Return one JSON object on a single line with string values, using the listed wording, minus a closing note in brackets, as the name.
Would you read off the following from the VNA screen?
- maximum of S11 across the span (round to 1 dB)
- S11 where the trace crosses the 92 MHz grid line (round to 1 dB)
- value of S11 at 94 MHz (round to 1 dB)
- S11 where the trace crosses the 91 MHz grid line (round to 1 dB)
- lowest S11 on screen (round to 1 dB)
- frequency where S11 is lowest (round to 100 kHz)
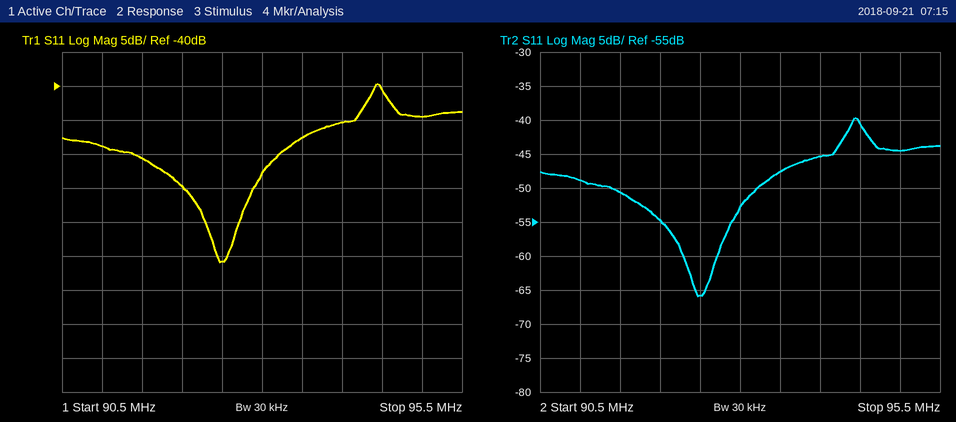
{"maximum of S11 across the span": "-40 dB", "S11 where the trace crosses the 92 MHz grid line": "-55 dB", "value of S11 at 94 MHz": "-45 dB", "S11 where the trace crosses the 91 MHz grid line": "-49 dB", "lowest S11 on screen": "-66 dB", "frequency where S11 is lowest": "92.5 MHz"}
